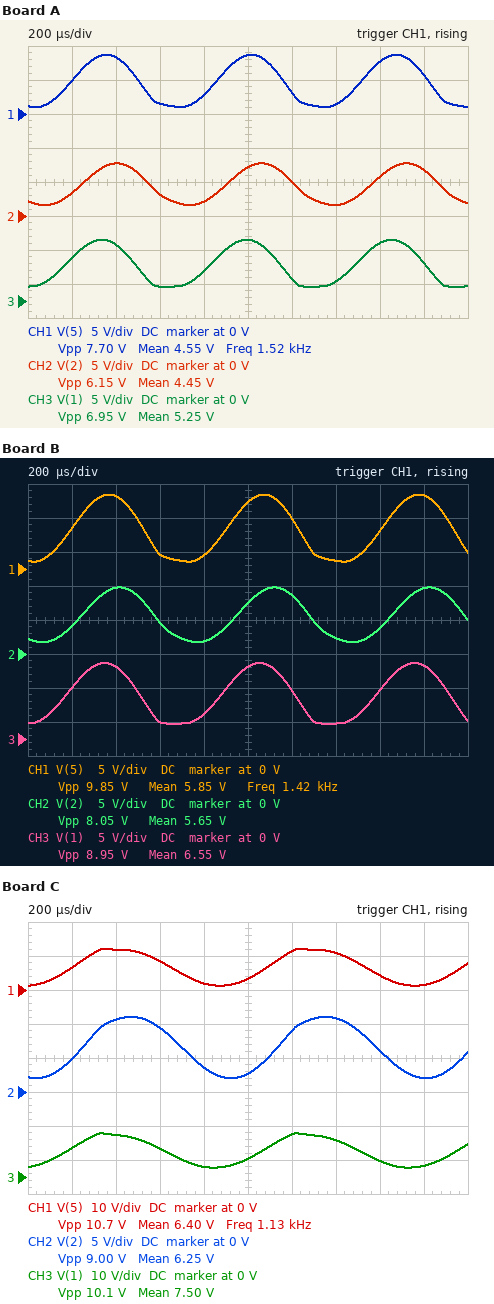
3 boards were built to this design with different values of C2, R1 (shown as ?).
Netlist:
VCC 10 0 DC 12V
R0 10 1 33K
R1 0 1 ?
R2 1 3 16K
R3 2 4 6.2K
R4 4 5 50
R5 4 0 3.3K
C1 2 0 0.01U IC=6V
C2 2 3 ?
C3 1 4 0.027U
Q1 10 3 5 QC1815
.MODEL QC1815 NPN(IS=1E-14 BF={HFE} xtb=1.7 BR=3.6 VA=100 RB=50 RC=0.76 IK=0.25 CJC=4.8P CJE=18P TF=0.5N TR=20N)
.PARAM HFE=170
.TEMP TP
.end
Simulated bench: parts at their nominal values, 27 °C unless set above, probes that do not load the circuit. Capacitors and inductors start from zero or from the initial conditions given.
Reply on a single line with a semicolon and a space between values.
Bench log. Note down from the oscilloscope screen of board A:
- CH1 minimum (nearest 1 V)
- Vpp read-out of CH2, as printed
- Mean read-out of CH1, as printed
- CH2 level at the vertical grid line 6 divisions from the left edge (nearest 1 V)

1 V; 6.15 V; 4.55 V; 5 V
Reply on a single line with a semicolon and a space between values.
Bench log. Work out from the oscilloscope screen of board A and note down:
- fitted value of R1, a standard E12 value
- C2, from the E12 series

27 kΩ; 3.3 nF
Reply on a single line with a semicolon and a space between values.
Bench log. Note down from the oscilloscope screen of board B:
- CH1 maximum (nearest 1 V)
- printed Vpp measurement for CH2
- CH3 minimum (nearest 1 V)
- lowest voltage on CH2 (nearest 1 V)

11 V; 8.05 V; 2 V; 2 V
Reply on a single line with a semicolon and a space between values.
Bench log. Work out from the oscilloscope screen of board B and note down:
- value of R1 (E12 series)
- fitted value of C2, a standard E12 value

39 kΩ; 3.3 nF
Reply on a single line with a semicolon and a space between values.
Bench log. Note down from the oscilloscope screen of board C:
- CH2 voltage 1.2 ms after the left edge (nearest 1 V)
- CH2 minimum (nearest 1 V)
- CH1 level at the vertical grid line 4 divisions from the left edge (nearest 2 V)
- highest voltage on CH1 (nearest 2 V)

9 V; 2 V; 2 V; 12 V
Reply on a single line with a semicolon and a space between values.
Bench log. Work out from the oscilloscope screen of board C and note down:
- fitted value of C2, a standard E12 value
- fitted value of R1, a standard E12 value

5.6 nF; 68 kΩ
